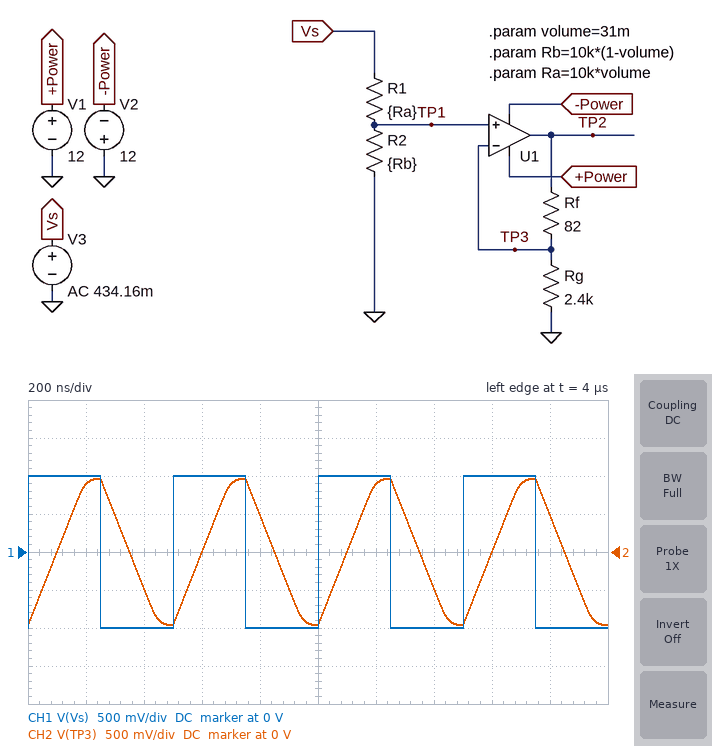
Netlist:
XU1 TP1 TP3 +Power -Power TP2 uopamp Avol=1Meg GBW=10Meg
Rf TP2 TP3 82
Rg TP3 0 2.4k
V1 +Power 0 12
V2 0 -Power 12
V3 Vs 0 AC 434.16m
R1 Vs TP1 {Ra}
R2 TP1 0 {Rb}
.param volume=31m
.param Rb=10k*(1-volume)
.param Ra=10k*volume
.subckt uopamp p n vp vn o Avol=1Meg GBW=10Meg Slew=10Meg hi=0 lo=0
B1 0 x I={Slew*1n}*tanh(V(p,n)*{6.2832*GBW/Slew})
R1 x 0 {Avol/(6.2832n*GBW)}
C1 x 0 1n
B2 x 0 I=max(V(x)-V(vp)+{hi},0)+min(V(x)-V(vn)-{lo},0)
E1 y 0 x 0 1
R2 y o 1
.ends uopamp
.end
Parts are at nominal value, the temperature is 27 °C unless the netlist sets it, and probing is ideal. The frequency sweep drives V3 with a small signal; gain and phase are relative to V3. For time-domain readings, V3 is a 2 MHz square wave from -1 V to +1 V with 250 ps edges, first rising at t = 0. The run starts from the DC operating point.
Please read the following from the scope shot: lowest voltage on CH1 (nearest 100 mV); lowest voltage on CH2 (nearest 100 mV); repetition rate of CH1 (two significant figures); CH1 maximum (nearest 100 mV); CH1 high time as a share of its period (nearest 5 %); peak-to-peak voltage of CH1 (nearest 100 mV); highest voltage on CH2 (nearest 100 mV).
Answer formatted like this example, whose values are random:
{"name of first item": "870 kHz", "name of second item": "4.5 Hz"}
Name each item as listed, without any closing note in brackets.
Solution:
{"lowest voltage on CH1": "-1.0 V", "lowest voltage on CH2": "-1.0 V", "repetition rate of CH1": "2.0 MHz", "CH1 maximum": "1.0 V", "CH1 high time as a share of its period": "50 %", "peak-to-peak voltage of CH1": "2.0 V", "highest voltage on CH2": "1.0 V"}
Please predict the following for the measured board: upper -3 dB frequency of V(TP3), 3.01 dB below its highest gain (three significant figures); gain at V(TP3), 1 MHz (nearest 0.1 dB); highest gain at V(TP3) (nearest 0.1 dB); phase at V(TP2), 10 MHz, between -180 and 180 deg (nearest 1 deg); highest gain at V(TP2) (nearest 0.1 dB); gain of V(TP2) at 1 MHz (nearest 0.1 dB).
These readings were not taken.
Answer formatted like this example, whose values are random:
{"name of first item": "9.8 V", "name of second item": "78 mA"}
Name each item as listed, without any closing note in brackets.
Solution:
{"upper -3 dB frequency of V(TP3), 3.01 dB below its highest gain": "9.67 MHz", "gain at V(TP3), 1 MHz": "-0.3 dB", "highest gain at V(TP3)": "-0.3 dB", "phase at V(TP2), 10 MHz, between -180 and 180 deg": "-46 deg", "highest gain at V(TP2)": "0 dB", "gain of V(TP2) at 1 MHz": "0 dB"}
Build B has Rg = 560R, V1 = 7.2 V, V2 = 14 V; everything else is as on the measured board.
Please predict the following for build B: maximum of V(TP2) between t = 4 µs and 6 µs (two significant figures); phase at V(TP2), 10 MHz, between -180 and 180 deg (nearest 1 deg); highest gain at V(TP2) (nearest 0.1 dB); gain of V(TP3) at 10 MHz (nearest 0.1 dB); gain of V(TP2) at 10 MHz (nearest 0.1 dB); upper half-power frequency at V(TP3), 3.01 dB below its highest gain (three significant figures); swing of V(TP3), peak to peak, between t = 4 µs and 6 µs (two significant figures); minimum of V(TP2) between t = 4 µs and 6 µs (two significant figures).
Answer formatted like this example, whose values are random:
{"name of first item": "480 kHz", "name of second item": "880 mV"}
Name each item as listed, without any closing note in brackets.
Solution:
{"maximum of V(TP2) between t = 4 µs and 6 µs": "1.1 V", "phase at V(TP2), 10 MHz, between -180 and 180 deg": "-49 deg", "highest gain at V(TP2)": "0.9 dB", "gain of V(TP3) at 10 MHz": "-3.9 dB", "gain of V(TP2) at 10 MHz": "-2.7 dB", "upper half-power frequency at V(TP3), 3.01 dB below its highest gain": "8.71 MHz", "swing of V(TP3), peak to peak, between t = 4 µs and 6 µs": "1.9 V", "minimum of V(TP2) between t = 4 µs and 6 µs": "-1.1 V"}
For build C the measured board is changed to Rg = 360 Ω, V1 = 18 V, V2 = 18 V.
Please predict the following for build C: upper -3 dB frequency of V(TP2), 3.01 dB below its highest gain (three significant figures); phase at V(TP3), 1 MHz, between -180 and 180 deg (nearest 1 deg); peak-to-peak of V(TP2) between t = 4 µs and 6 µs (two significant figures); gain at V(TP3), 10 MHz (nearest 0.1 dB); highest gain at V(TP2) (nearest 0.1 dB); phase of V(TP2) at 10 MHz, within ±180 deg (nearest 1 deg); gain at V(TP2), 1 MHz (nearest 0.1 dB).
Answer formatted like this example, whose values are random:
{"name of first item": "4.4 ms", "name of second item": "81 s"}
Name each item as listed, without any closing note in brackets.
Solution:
{"upper -3 dB frequency of V(TP2), 3.01 dB below its highest gain": "8.13 MHz", "phase at V(TP3), 1 MHz, between -180 and 180 deg": "-7 deg", "peak-to-peak of V(TP2) between t = 4 µs and 6 µs": "2.3 V", "gain at V(TP3), 10 MHz": "-4.3 dB", "highest gain at V(TP2)": "1.5 dB", "phase of V(TP2) at 10 MHz, within ±180 deg": "-51 deg", "gain at V(TP2), 1 MHz": "1.4 dB"}
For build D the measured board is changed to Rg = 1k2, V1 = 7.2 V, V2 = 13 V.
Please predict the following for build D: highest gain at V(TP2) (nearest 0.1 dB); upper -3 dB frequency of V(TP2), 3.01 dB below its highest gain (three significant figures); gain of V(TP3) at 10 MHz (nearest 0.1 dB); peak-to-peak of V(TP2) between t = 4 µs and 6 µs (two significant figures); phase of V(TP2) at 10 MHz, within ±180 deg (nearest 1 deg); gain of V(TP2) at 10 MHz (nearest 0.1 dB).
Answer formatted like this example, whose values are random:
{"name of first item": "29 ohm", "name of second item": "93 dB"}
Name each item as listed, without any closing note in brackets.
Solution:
{"highest gain at V(TP2)": "0.3 dB", "upper -3 dB frequency of V(TP2), 3.01 dB below its highest gain": "9.35 MHz", "gain of V(TP3) at 10 MHz": "-3.6 dB", "peak-to-peak of V(TP2) between t = 4 µs and 6 µs": "2.1 V", "phase of V(TP2) at 10 MHz, within ±180 deg": "-47 deg", "gain of V(TP2) at 10 MHz": "-3.0 dB"}
